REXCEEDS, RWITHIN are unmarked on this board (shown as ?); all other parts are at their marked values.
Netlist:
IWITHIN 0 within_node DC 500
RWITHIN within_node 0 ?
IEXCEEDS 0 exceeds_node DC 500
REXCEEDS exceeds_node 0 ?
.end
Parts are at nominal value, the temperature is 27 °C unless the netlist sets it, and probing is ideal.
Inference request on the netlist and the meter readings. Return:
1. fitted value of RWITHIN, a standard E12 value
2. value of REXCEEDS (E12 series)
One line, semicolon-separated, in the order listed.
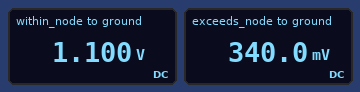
2.2 mΩ; 680 µΩ
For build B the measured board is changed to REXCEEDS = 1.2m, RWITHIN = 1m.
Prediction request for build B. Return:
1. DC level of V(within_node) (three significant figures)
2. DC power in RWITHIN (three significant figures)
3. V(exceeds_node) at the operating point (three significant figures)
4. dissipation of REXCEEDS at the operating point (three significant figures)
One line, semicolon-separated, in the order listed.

500 mV; 250 W; 600 mV; 300 W
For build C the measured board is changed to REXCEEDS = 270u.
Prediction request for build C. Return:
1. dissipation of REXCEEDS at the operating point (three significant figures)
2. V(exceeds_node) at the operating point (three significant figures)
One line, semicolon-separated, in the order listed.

67.5 W; 135 mV
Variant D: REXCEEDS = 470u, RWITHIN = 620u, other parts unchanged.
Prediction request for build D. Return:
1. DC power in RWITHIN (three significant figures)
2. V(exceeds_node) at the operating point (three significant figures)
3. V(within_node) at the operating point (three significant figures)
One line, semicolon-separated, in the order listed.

155 W; 235 mV; 310 mV
